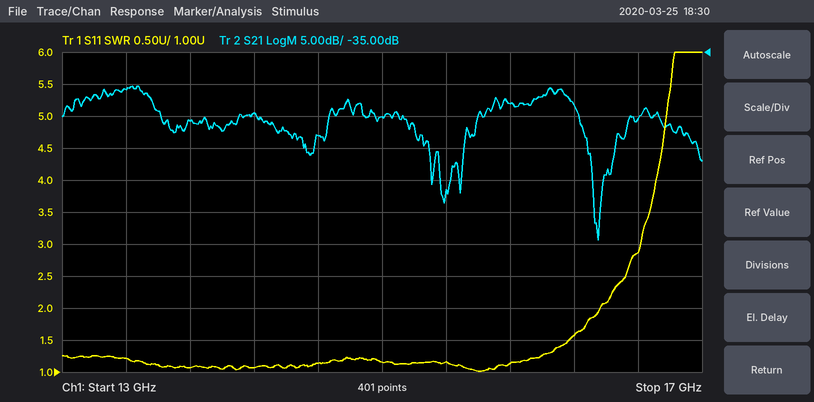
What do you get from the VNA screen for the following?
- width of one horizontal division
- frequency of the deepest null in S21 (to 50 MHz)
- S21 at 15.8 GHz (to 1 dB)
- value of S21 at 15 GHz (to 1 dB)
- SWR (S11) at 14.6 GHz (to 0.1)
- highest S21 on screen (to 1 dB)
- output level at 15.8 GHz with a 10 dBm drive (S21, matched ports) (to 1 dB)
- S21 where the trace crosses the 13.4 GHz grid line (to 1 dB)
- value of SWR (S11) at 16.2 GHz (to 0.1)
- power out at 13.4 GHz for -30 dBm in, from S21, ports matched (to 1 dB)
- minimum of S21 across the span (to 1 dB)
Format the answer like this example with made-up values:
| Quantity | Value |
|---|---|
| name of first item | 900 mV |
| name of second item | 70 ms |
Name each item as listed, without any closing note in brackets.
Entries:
| Quantity | Value |
|---|---|
| width of one horizontal division | 400 MHz |
| frequency of the deepest null in S21 | 16.35 GHz |
| S21 at 15.8 GHz | -43 dB |
| value of S21 at 15 GHz | -45 dB |
| SWR (S11) at 14.6 GHz | 1.1 |
| highest S21 on screen | -40 dB |
| output level at 15.8 GHz with a 10 dBm drive (S21, matched ports) | -33 dBm |
| S21 where the trace crosses the 13.4 GHz grid line | -41 dB |
| value of SWR (S11) at 16.2 GHz | 1.6 |
| power out at 13.4 GHz for -30 dBm in, from S21, ports matched | -71 dBm |
| minimum of S21 across the span | -64 dB |
